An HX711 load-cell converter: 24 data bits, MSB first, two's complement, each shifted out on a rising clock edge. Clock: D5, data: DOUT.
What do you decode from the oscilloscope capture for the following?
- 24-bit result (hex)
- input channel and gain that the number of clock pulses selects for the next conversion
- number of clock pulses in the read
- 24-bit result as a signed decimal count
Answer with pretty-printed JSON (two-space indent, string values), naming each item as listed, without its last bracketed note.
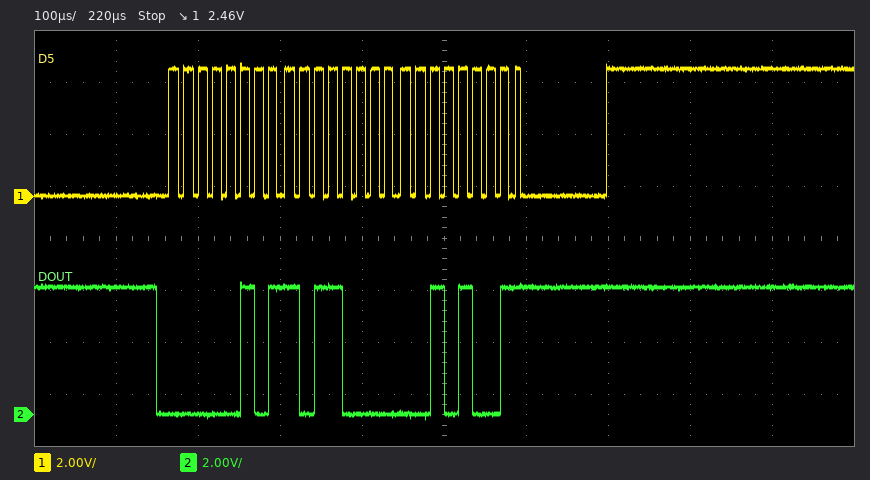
{
  "24-bit result": "0x05B029",
  "input channel and gain that the number of clock pulses selects for the next conversion": "channel B, gain 32",
  "number of clock pulses in the read": "26",
  "24-bit result as a signed decimal count": "372777"
}
